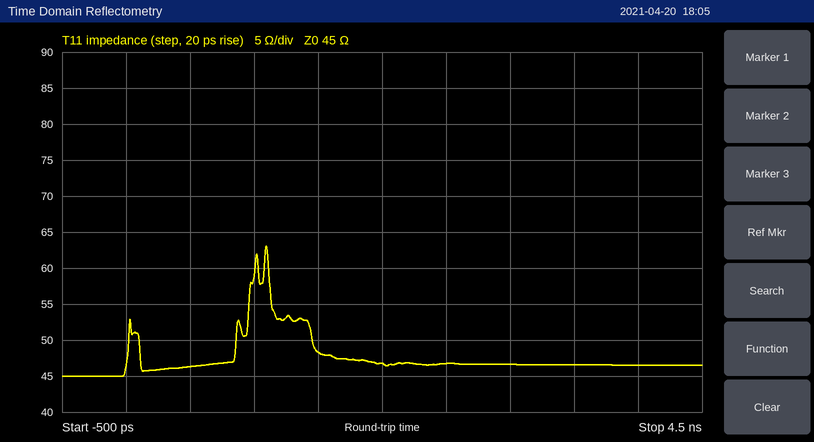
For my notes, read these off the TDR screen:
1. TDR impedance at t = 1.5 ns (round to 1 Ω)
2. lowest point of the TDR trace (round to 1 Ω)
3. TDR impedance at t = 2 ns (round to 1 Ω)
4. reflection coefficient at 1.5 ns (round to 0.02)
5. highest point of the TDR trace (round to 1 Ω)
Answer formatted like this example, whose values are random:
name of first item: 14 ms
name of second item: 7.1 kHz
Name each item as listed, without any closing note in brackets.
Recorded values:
TDR impedance at t = 1.5 ns: 48 Ω
lowest point of the TDR trace: 45 Ω
TDR impedance at t = 2 ns: 47 Ω
reflection coefficient at 1.5 ns: +0.04
highest point of the TDR trace: 63 Ω
